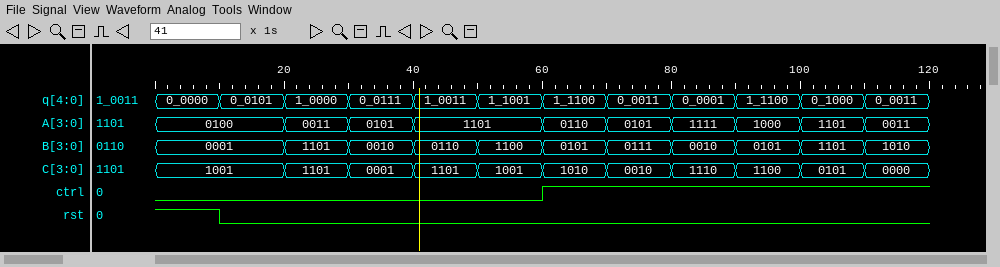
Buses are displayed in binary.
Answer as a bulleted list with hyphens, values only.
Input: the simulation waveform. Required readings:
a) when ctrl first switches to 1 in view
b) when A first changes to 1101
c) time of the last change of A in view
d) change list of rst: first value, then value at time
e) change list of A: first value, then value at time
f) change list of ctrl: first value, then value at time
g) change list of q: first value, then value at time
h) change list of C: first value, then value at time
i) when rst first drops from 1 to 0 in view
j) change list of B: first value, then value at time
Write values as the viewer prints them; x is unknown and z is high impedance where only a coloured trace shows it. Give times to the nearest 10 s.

- 60 s
- 40 s
- 110 s
- 1, 0 at 10 s
- 0100, 0011 at 20 s, 0101 at 30 s, 1101 at 40 s, 0110 at 60 s, 0101 at 70 s, 1111 at 80 s, 1000 at 90 s, 1101 at 100 s, 0011 at 110 s
- 0, 1 at 60 s
- 0_0000, 0_0101 at 10 s, 1_0000 at 20 s, 0_0111 at 30 s, 1_0011 at 40 s, 1_1001 at 50 s, 1_1100 at 60 s, 0_0011 at 70 s, 0_0001 at 80 s, 1_1100 at 90 s, 0_1000 at 100 s, 0_0011 at 110 s
- 1001, 1101 at 20 s, 0001 at 30 s, 1101 at 40 s, 1001 at 50 s, 1010 at 60 s, 0010 at 70 s, 1110 at 80 s, 1100 at 90 s, 0101 at 100 s, 0000 at 110 s
- 10 s
- 0001, 1101 at 20 s, 0010 at 30 s, 0110 at 40 s, 1100 at 50 s, 0101 at 60 s, 0111 at 70 s, 0010 at 80 s, 0101 at 90 s, 1101 at 100 s, 1010 at 110 s
